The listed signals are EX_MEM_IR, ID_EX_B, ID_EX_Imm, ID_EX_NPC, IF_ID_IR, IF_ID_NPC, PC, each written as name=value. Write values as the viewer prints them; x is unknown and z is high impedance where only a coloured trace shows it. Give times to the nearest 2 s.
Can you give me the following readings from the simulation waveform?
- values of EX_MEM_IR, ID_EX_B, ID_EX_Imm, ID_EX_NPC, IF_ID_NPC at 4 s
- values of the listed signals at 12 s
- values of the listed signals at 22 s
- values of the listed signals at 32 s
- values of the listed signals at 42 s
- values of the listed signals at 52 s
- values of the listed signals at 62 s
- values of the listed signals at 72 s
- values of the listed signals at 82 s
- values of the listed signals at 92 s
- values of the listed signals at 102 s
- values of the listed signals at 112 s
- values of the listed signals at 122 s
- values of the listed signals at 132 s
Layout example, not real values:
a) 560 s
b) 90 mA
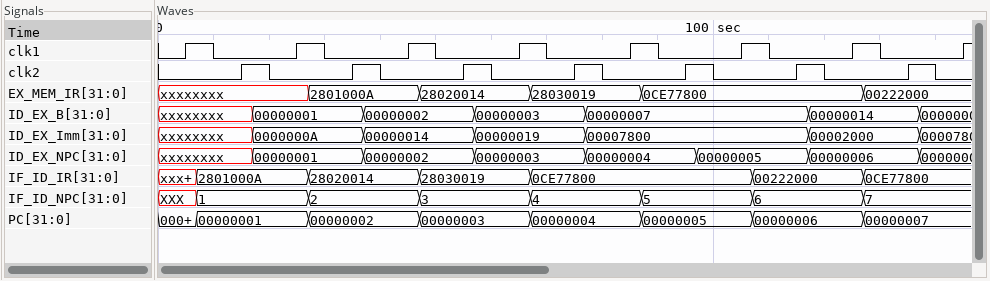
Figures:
a) EX_MEM_IR=xxxxxxxx, ID_EX_B=xxxxxxxx, ID_EX_Imm=xxxxxxxx, ID_EX_NPC=xxxxxxxx, IF_ID_NPC=XXX
b) EX_MEM_IR=xxxxxxxx, ID_EX_B=xxxxxxxx, ID_EX_Imm=xxxxxxxx, ID_EX_NPC=xxxxxxxx, IF_ID_IR=2801000A, IF_ID_NPC=1, PC=00000001
c) EX_MEM_IR=xxxxxxxx, ID_EX_B=00000001, ID_EX_Imm=0000000A, ID_EX_NPC=00000001, IF_ID_IR=2801000A, IF_ID_NPC=1, PC=00000001
d) EX_MEM_IR=2801000A, ID_EX_B=00000001, ID_EX_Imm=0000000A, ID_EX_NPC=00000001, IF_ID_IR=28020014, IF_ID_NPC=2, PC=00000002
e) EX_MEM_IR=2801000A, ID_EX_B=00000002, ID_EX_Imm=00000014, ID_EX_NPC=00000002, IF_ID_IR=28020014, IF_ID_NPC=2, PC=00000002
f) EX_MEM_IR=28020014, ID_EX_B=00000002, ID_EX_Imm=00000014, ID_EX_NPC=00000002, IF_ID_IR=28030019, IF_ID_NPC=3, PC=00000003
g) EX_MEM_IR=28020014, ID_EX_B=00000003, ID_EX_Imm=00000019, ID_EX_NPC=00000003, IF_ID_IR=28030019, IF_ID_NPC=3, PC=00000003
h) EX_MEM_IR=28030019, ID_EX_B=00000003, ID_EX_Imm=00000019, ID_EX_NPC=00000003, IF_ID_IR=0CE77800, IF_ID_NPC=4, PC=00000004
i) EX_MEM_IR=28030019, ID_EX_B=00000007, ID_EX_Imm=00007800, ID_EX_NPC=00000004, IF_ID_IR=0CE77800, IF_ID_NPC=4, PC=00000004
j) EX_MEM_IR=0CE77800, ID_EX_B=00000007, ID_EX_Imm=00007800, ID_EX_NPC=00000004, IF_ID_IR=0CE77800, IF_ID_NPC=5, PC=00000005
k) EX_MEM_IR=0CE77800, ID_EX_B=00000007, ID_EX_Imm=00007800, ID_EX_NPC=00000005, IF_ID_IR=0CE77800, IF_ID_NPC=5, PC=00000005
l) EX_MEM_IR=0CE77800, ID_EX_B=00000007, ID_EX_Imm=00007800, ID_EX_NPC=00000005, IF_ID_IR=00222000, IF_ID_NPC=6, PC=00000006
m) EX_MEM_IR=0CE77800, ID_EX_B=00000014, ID_EX_Imm=00002000, ID_EX_NPC=00000006, IF_ID_IR=00222000, IF_ID_NPC=6, PC=00000006
n) EX_MEM_IR=00222000, ID_EX_B=00000014, ID_EX_Imm=00002000, ID_EX_NPC=00000006, IF_ID_IR=0CE77800, IF_ID_NPC=7, PC=00000007
